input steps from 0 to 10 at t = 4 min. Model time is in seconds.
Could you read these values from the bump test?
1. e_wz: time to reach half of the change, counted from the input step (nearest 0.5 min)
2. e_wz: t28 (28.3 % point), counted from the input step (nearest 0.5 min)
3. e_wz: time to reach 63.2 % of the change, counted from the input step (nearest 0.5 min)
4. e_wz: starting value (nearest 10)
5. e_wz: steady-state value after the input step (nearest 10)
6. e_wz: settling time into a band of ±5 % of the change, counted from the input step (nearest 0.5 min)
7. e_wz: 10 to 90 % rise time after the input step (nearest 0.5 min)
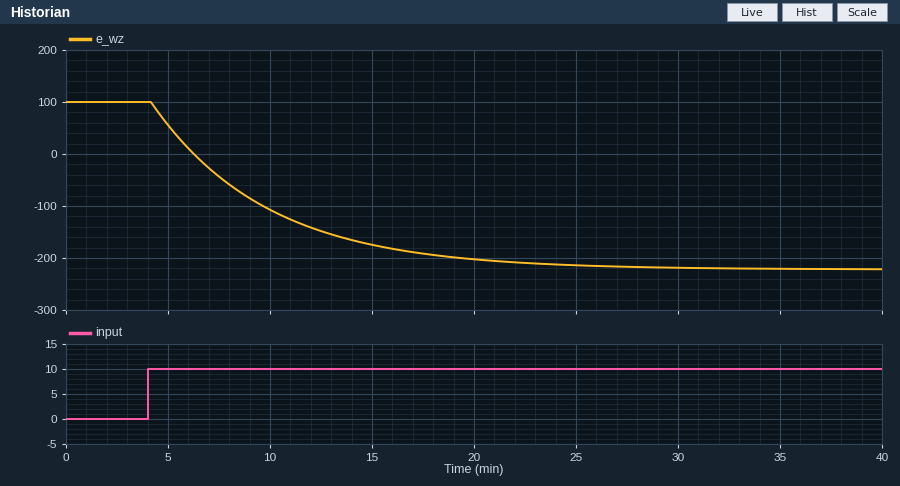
4.0 min
2.0 min
6.0 min
100
-220
17.0 min
12.5 min
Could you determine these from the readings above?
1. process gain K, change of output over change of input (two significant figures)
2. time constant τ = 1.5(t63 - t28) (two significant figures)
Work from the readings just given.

-32
6.0 min
